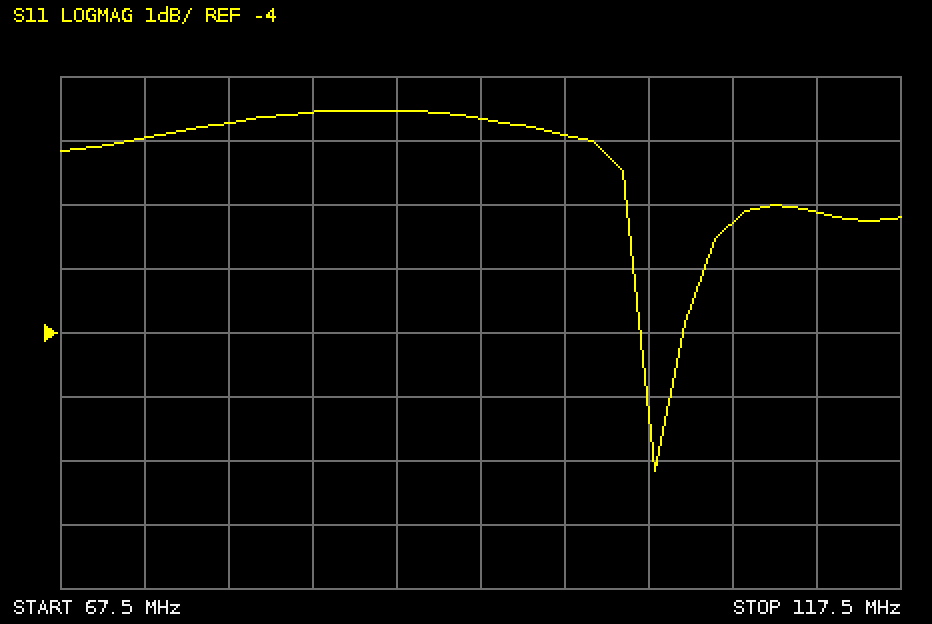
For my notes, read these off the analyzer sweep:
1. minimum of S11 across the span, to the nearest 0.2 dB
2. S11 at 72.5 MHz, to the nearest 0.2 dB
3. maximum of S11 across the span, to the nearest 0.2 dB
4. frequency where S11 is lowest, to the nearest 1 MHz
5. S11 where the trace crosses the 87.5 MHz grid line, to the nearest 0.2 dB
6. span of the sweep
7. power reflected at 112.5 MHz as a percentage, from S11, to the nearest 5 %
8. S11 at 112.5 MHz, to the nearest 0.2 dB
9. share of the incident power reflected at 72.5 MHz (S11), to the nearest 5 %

-6.2 dB
-1.0 dB
-0.6 dB
103 MHz
-0.6 dB
50 MHz
60 %
-2.2 dB
80 %
